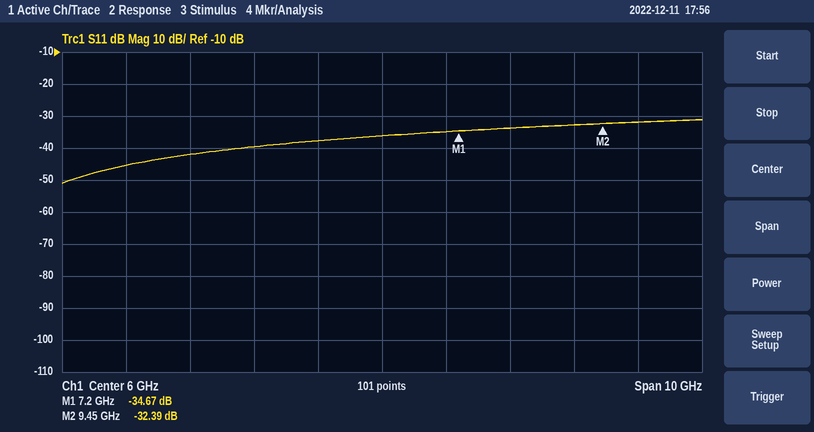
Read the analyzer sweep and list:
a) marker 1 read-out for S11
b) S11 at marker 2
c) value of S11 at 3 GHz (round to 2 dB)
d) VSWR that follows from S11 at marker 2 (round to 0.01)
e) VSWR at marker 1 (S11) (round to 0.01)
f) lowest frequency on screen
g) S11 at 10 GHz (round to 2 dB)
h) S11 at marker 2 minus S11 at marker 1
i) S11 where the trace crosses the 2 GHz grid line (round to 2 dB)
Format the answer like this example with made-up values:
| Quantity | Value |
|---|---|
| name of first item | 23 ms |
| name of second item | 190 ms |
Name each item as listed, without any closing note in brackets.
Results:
| Quantity | Value |
|---|---|
| marker 1 read-out for S11 | -34.67 dB |
| S11 at marker 2 | -32.39 dB |
| value of S11 at 3 GHz | -42 dB |
| VSWR that follows from S11 at marker 2 | 1.05 |
| VSWR at marker 1 (S11) | 1.04 |
| lowest frequency on screen | 1 GHz |
| S11 at 10 GHz | -32 dB |
| S11 at marker 2 minus S11 at marker 1 | 2.28 dB |
| S11 where the trace crosses the 2 GHz grid line | -46 dB |
